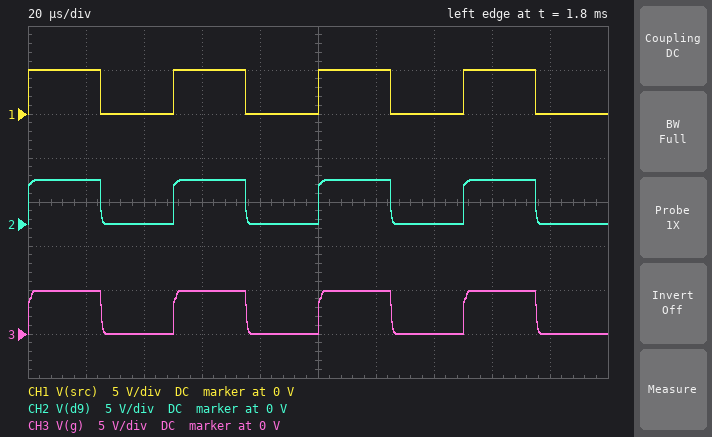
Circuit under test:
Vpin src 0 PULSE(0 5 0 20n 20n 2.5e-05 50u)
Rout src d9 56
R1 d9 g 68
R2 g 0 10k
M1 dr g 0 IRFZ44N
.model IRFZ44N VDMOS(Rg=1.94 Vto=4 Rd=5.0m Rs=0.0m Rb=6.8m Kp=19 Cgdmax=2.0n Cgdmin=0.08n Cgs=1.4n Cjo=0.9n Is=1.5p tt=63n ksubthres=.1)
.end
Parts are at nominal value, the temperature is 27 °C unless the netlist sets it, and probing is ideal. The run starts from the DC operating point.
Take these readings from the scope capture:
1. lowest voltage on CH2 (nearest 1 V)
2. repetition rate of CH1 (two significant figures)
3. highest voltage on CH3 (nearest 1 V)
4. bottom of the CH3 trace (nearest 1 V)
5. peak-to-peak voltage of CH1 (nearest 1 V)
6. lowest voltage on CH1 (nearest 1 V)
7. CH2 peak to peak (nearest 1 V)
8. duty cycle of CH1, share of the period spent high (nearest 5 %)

0 V
20 kHz
5 V
0 V
5 V
0 V
5 V
50 %
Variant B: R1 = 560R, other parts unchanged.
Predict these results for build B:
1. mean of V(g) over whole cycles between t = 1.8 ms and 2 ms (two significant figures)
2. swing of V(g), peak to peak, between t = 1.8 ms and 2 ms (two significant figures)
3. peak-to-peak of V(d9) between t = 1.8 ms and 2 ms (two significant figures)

2.4 V
4.7 V
5.0 V
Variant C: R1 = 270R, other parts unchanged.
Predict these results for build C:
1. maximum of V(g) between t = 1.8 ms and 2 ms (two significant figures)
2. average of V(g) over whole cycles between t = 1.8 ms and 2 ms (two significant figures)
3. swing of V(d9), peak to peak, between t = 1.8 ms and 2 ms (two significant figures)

4.8 V
2.4 V
5.0 V
